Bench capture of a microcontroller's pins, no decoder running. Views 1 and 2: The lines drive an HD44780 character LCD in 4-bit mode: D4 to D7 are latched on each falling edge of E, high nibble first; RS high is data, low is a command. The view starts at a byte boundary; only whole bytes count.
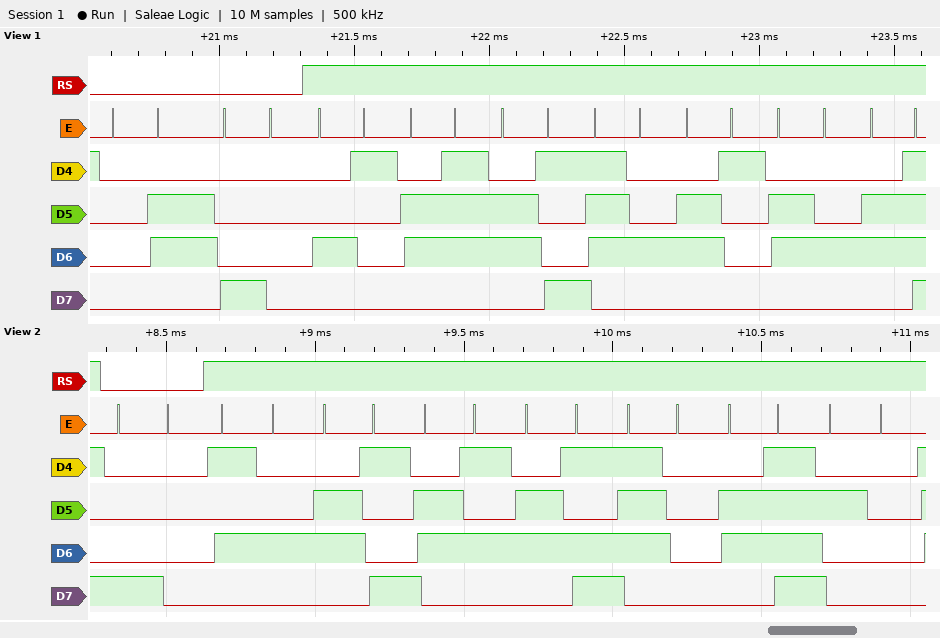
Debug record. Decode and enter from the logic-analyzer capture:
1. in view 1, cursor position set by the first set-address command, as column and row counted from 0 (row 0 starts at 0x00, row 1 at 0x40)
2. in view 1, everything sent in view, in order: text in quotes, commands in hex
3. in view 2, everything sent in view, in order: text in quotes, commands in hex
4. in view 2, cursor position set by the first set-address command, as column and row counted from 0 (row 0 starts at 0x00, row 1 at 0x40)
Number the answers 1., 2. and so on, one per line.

1. column 0, row 0
2. 0x06 0x80 "Agitado"
3. 0x80 "Tiempo "
4. column 0, row 0
